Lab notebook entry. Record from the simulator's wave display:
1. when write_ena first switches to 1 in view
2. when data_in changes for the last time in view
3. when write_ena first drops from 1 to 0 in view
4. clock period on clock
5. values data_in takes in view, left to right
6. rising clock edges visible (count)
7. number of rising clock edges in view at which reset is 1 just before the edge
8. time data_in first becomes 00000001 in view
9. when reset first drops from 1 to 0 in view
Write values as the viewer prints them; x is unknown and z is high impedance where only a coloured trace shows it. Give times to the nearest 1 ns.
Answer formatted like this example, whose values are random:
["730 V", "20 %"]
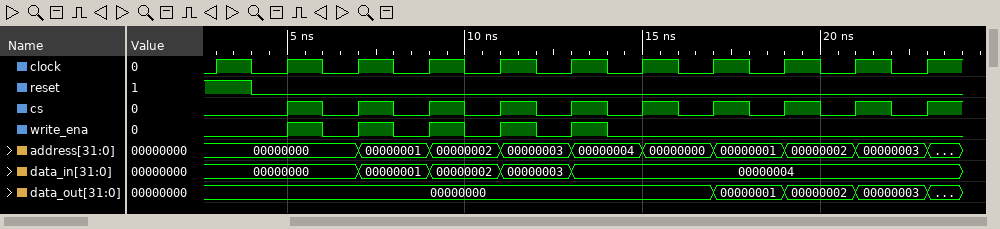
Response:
["5 ns", "13 ns", "6 ns", "2 ns", "00000000, 00000001, 00000002, 00000003, 00000004", "11", "1", "7 ns", "4 ns"]
